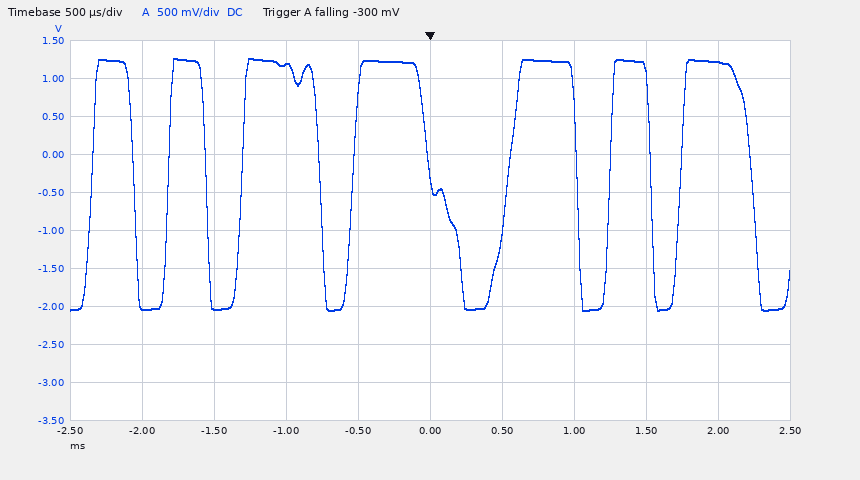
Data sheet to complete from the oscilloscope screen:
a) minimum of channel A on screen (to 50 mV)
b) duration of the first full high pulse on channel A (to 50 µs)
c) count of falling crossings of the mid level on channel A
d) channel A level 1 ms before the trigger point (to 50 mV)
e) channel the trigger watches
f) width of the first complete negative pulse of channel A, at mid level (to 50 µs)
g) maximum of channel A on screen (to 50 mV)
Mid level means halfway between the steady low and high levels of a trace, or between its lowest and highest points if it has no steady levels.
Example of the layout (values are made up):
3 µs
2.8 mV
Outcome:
-2.05 V
300 µs
7
1.20 V
channel A
250 µs
1.25 V
